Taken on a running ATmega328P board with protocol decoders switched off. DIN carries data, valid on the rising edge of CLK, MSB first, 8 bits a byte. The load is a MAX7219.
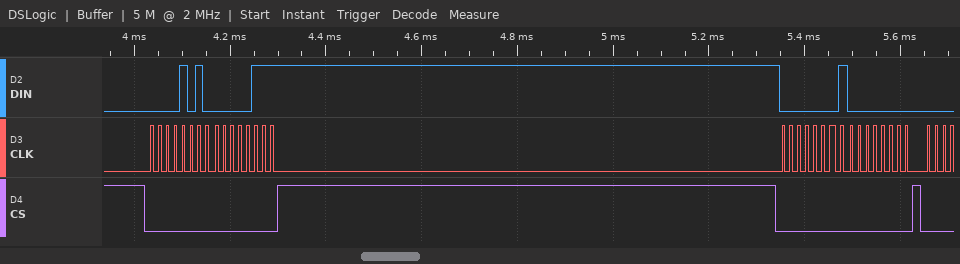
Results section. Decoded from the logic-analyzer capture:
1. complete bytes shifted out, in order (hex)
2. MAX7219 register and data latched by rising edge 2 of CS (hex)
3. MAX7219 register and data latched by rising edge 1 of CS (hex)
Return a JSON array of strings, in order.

["0A 07 01 00", "register 0x1, data 0x00", "register 0xA, data 0x07"]
